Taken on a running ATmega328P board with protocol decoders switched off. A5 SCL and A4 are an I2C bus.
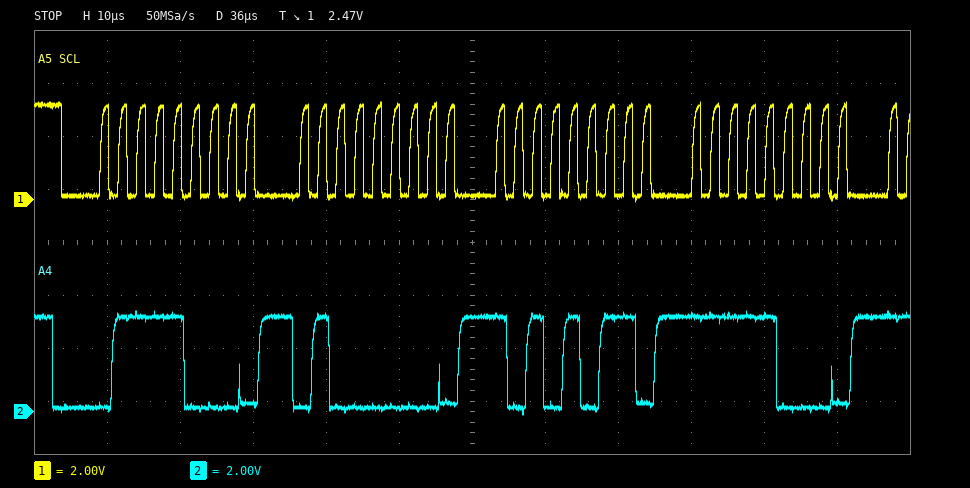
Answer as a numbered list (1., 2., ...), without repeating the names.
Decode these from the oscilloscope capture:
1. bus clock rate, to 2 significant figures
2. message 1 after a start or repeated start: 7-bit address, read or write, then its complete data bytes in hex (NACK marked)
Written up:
1. 400 kHz
2. 0x3C write: 40 AB F8
